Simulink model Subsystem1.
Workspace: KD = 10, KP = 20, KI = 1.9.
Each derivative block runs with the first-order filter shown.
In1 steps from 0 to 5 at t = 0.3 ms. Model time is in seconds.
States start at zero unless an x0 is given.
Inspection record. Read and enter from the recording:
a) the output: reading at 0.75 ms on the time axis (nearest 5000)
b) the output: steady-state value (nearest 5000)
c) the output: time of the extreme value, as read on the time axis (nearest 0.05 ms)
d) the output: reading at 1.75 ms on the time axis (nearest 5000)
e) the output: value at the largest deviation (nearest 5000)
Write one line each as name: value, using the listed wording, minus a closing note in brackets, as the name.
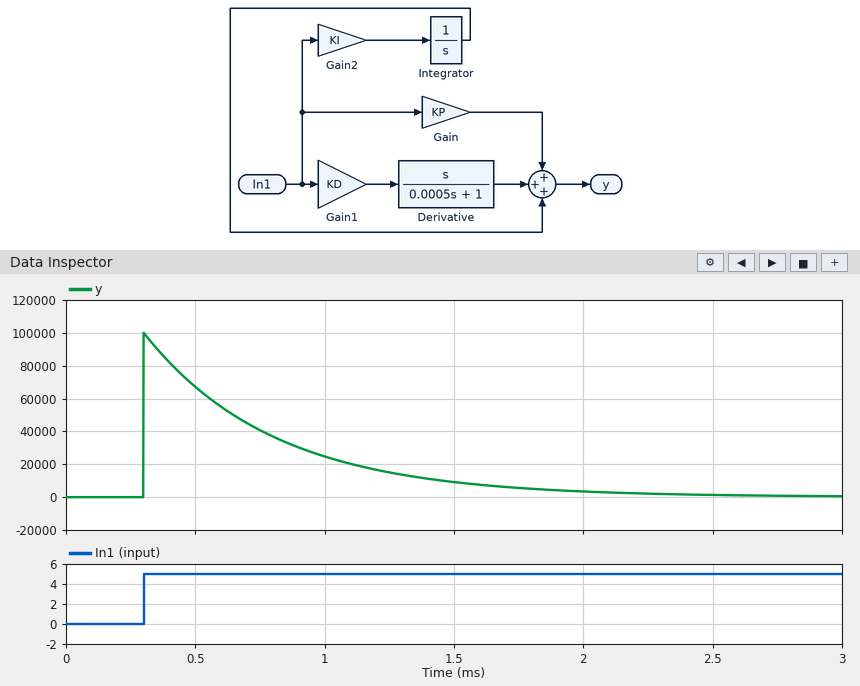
the output: reading at 0.75 ms on the time axis: 40000
the output: steady-state value: 0
the output: time of the extreme value, as read on the time axis: 0.30 ms
the output: reading at 1.75 ms on the time axis: 5000
the output: value at the largest deviation: 100000
